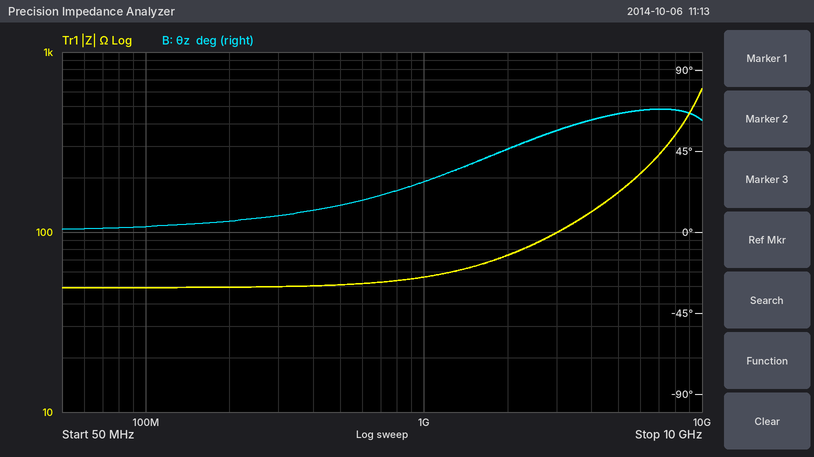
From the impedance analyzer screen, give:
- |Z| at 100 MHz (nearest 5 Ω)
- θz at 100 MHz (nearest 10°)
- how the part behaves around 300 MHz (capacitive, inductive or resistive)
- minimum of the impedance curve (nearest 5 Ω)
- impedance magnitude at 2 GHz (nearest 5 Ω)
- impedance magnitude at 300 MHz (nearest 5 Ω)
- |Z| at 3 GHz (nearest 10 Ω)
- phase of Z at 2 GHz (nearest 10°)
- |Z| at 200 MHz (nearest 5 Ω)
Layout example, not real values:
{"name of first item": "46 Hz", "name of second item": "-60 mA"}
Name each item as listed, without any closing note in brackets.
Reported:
{"|Z| at 100 MHz": "50 Ω", "θz at 100 MHz": "0°", "how the part behaves around 300 MHz": "resistive", "minimum of the impedance curve": "50 Ω", "impedance magnitude at 2 GHz": "75 Ω", "impedance magnitude at 300 MHz": "50 Ω", "|Z| at 3 GHz": "100 Ω", "phase of Z at 2 GHz": "50°", "|Z| at 200 MHz": "50 Ω"}
